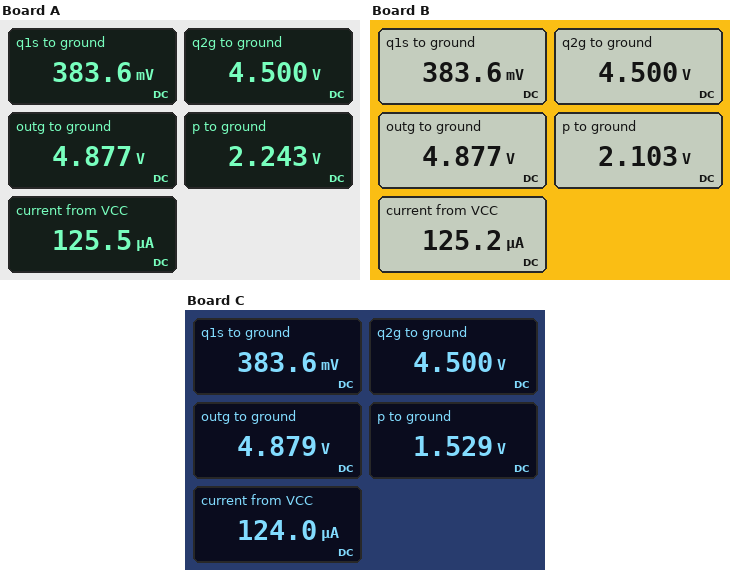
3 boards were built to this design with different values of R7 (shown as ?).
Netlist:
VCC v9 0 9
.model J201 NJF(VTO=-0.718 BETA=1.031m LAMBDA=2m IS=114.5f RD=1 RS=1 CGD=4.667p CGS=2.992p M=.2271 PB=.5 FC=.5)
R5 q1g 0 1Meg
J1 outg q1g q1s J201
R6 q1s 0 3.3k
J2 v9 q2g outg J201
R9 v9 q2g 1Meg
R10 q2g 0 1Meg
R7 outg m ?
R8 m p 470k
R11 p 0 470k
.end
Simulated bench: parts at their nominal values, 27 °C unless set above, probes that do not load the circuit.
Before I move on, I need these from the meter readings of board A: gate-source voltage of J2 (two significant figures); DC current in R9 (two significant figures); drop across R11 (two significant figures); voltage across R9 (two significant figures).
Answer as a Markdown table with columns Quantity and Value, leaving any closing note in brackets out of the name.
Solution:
| Quantity | Value |
|---|---|
| gate-source voltage of J2 | -380 mV |
| DC current in R9 | 4.5 µA |
| drop across R11 | 2.2 V |
| voltage across R9 | 4.5 V |
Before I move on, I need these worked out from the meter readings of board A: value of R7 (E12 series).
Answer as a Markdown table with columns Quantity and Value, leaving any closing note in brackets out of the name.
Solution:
| Quantity | Value |
|---|---|
| value of R7 | 82 kΩ |
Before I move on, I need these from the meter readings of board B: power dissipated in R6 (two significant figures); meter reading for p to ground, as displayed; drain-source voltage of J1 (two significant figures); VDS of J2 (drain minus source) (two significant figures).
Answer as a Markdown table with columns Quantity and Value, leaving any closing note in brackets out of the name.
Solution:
| Quantity | Value |
|---|---|
| power dissipated in R6 | 45 µW |
| meter reading for p to ground, as displayed | 2.103 V |
| drain-source voltage of J1 | 4.5 V |
| VDS of J2 (drain minus source) | 4.1 V |
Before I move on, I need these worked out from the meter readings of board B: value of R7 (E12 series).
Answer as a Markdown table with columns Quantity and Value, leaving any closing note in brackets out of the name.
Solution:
| Quantity | Value |
|---|---|
| value of R7 | 150 kΩ |
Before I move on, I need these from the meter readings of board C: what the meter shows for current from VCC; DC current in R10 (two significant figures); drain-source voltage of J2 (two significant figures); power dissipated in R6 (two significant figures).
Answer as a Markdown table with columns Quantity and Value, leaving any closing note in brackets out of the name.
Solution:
| Quantity | Value |
|---|---|
| what the meter shows for current from VCC | 124.0 µA |
| DC current in R10 | 4.5 µA |
| drain-source voltage of J2 | 4.1 V |
| power dissipated in R6 | 45 µW |
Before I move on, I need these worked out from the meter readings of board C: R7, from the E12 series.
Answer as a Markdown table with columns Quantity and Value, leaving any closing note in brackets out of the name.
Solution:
| Quantity | Value |
|---|---|
| R7, from the E12 series | 560 kΩ |
